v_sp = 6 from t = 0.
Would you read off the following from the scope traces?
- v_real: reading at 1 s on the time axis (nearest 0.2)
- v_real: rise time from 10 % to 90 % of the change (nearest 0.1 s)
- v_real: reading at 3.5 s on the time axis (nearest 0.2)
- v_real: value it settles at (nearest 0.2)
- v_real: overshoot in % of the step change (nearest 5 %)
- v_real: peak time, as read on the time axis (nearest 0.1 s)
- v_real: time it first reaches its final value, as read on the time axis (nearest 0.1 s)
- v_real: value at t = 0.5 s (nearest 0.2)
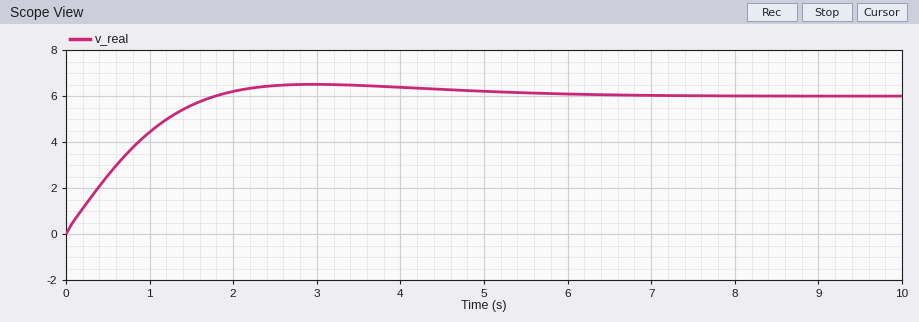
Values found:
4.4
1.3 s
6.4
6.0
10 %
3.0 s
1.8 s
2.6
